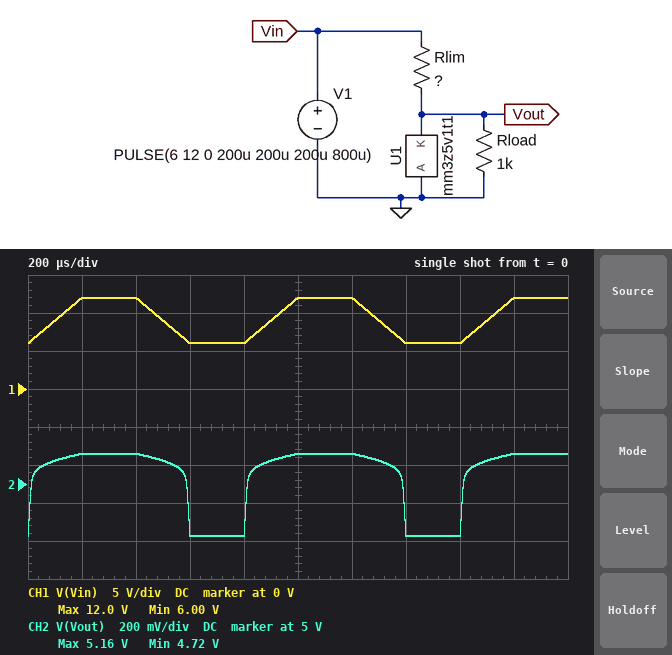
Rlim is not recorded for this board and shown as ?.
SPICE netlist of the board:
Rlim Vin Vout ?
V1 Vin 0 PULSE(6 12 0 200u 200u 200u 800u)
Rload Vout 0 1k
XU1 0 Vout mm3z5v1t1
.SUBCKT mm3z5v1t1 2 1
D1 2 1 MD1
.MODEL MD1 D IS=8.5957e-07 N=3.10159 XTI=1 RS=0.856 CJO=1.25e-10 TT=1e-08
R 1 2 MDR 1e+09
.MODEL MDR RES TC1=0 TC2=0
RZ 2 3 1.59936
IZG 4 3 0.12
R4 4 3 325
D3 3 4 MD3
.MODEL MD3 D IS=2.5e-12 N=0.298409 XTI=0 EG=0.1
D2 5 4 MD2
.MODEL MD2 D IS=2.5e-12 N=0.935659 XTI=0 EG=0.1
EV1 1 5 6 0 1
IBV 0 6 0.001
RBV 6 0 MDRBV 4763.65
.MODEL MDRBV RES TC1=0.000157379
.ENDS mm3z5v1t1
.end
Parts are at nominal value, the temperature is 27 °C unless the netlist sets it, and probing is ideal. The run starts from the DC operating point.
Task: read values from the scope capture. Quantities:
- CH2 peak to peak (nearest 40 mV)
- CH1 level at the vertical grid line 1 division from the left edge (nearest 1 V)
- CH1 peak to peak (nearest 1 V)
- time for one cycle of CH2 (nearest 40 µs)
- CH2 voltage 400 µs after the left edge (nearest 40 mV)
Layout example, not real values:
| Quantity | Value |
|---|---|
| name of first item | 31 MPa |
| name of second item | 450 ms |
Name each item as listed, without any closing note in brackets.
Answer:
| Quantity | Value |
|---|---|
| CH2 peak to peak | 440 mV |
| CH1 level at the vertical grid line 1 division from the left edge | 12 V |
| CH1 peak to peak | 6 V |
| time for one cycle of CH2 | 800 µs |
| CH2 voltage 400 µs after the left edge | 5.16 V |
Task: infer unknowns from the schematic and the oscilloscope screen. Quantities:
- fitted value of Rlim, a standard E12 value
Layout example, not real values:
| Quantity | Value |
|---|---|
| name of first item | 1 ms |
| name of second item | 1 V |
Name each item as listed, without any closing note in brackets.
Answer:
| Quantity | Value |
|---|---|
| fitted value of Rlim, a standard E12 value | 270 Ω |
